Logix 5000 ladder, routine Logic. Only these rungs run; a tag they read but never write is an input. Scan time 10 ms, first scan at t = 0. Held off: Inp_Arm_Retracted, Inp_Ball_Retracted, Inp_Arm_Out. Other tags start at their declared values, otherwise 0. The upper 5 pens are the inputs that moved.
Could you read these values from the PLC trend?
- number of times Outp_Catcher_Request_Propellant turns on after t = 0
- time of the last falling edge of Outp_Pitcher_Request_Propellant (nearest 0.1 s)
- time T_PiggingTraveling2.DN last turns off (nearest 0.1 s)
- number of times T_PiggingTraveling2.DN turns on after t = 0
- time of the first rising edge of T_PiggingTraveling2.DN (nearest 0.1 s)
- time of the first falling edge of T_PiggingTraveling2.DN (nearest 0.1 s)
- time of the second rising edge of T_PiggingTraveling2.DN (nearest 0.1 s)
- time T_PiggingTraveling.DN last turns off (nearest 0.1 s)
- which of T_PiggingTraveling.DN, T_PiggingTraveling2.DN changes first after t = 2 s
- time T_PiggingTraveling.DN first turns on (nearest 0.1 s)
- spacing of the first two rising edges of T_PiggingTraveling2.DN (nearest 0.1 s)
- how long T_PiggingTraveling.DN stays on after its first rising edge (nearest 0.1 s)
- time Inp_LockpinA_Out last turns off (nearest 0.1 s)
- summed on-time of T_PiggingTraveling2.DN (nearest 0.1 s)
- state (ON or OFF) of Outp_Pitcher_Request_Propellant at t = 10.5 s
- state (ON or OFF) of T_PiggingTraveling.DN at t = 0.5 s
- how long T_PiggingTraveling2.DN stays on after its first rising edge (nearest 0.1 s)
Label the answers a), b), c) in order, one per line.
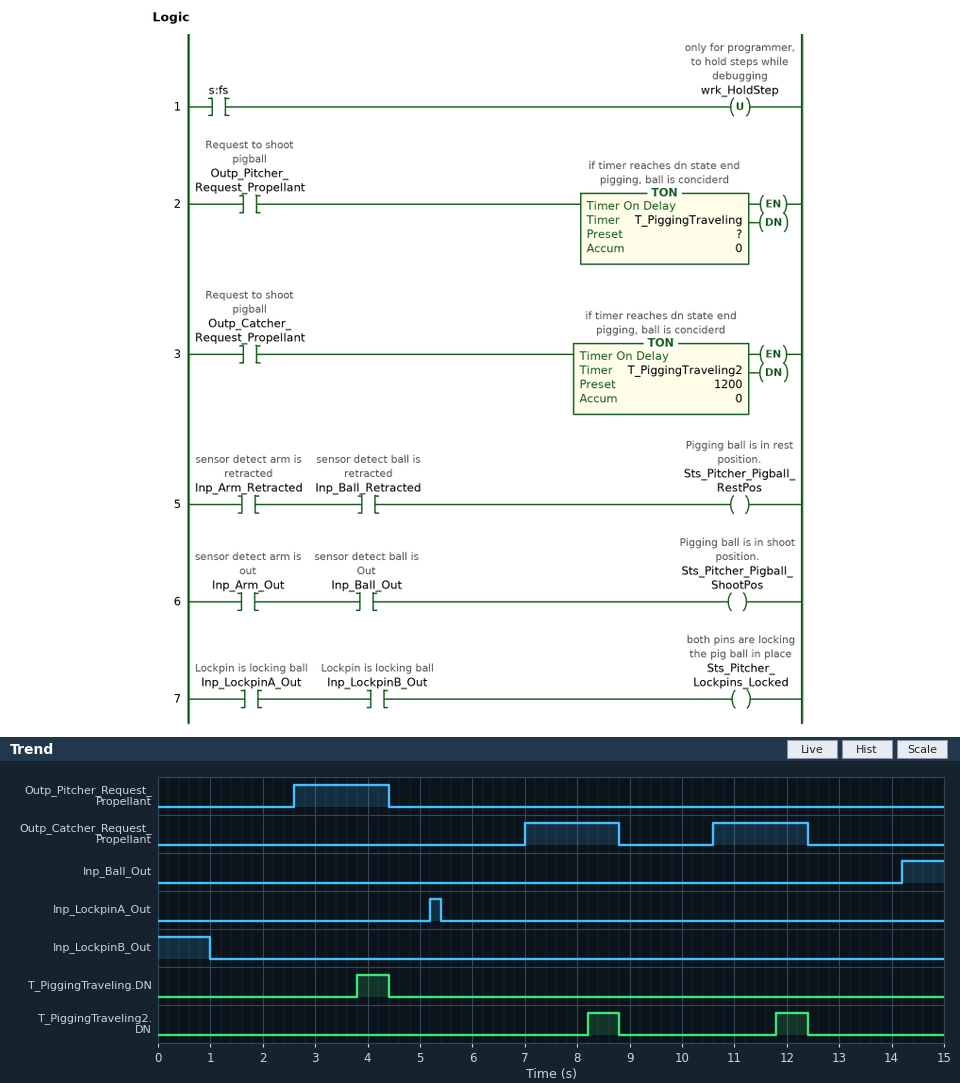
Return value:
a) 2
b) 4.4 s
c) 12.4 s
d) 2
e) 8.2 s
f) 8.8 s
g) 11.8 s
h) 4.4 s
i) T_PiggingTraveling.DN
j) 3.8 s
k) 3.6 s
l) 0.6 s
m) 5.4 s
n) 1.2 s
o) OFF
p) OFF
q) 0.6 s
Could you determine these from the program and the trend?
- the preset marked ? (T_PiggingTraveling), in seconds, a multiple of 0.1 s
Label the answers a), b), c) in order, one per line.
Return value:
a) 1.2 s
